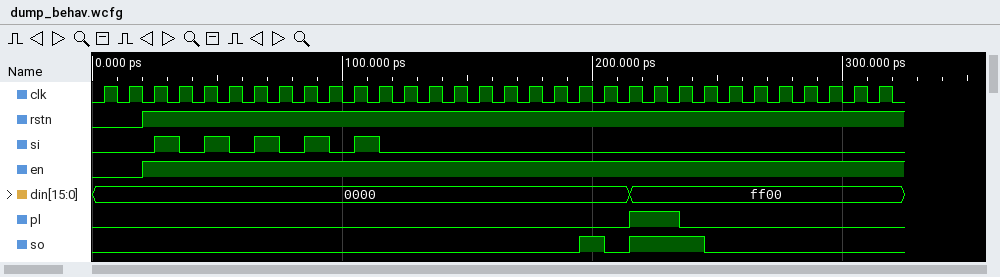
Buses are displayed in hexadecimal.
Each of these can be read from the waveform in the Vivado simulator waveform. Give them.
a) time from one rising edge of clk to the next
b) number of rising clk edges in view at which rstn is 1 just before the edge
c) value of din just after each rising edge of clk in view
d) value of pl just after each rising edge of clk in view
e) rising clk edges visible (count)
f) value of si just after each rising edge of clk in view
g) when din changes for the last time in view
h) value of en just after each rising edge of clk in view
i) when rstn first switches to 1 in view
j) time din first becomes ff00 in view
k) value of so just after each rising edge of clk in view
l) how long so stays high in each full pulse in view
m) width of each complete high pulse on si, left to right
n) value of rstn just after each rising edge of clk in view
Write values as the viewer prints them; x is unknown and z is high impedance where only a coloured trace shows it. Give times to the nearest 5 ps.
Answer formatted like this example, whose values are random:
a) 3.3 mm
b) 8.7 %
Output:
a) 10 ps
b) 30
c) 0000, 0000, 0000, 0000, 0000, 0000, 0000, 0000, 0000, 0000, 0000, 0000, 0000, 0000, 0000, 0000, 0000, 0000, 0000, 0000, 0000, ff00, ff00, ff00, ff00, ff00, ff00, ff00, ff00, ff00, ff00, ff00
d) 0 0 0 0 0 0 0 0 0 0 0 0 0 0 0 0 0 0 0 0 0 1 1 0 0 0 0 0 0 0 0 0
e) 32
f) 0 0 1 0 1 0 1 0 1 0 1 0 0 0 0 0 0 0 0 0 0 0 0 0 0 0 0 0 0 0 0 0
g) 215 ps
h) 0 0 1 1 1 1 1 1 1 1 1 1 1 1 1 1 1 1 1 1 1 1 1 1 1 1 1 1 1 1 1 1
i) 20 ps
j) 215 ps
k) 0 0 0 0 0 0 0 0 0 0 0 0 0 0 0 0 0 0 0 1 0 1 1 1 0 0 0 0 0 0 0 0
l) 10 ps, 30 ps
m) 10 ps, 10 ps, 10 ps, 10 ps, 10 ps
n) 0 0 1 1 1 1 1 1 1 1 1 1 1 1 1 1 1 1 1 1 1 1 1 1 1 1 1 1 1 1 1 1
